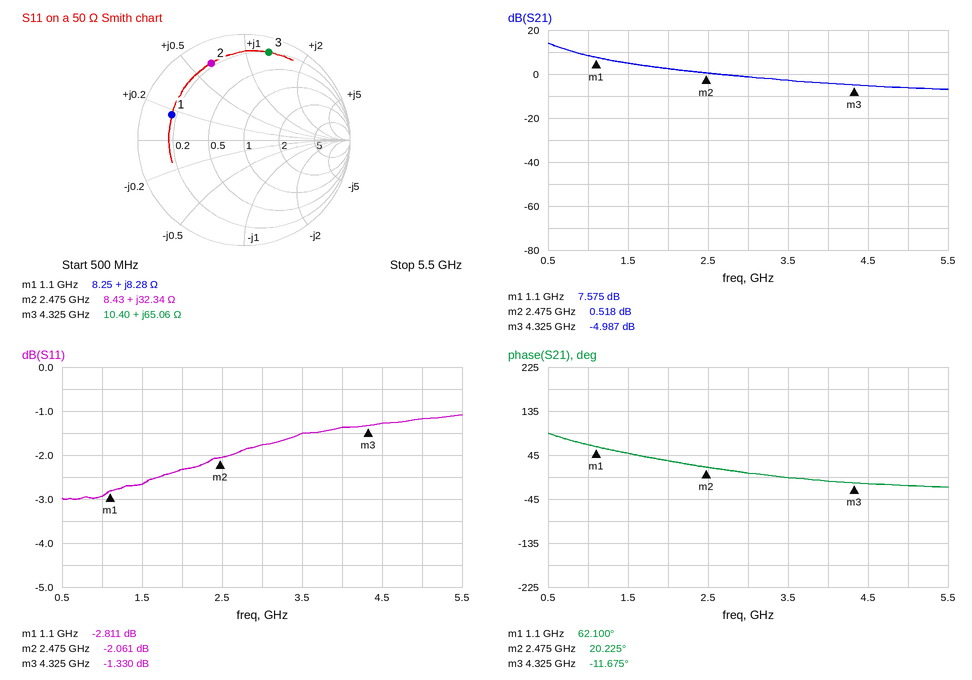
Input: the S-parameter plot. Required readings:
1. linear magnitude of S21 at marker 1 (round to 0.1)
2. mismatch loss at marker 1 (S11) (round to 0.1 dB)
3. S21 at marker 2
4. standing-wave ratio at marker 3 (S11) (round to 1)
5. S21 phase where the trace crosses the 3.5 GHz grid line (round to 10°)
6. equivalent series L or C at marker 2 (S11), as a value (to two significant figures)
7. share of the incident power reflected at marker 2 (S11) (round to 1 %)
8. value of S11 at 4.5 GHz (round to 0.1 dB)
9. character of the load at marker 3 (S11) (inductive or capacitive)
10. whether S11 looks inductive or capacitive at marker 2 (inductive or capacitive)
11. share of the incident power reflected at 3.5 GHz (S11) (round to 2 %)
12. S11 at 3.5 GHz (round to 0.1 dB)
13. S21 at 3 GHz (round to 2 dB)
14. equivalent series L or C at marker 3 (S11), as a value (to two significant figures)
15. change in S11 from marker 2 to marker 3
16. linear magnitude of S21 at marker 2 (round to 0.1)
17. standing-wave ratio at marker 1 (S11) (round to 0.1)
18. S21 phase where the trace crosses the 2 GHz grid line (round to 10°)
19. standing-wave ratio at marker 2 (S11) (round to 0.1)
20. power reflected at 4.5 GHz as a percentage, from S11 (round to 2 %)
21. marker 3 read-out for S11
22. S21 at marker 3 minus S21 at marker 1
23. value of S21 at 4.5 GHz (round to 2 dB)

2.4
3.2 dB
0.518 dB
13
0°
2.1 nH
62 %
-1.3 dB
inductive
inductive
70 %
-1.5 dB
-2 dB
2.4 nH
0.731 dB
1.1
6.2
30°
8.5
74 %
-1.330 dB
-12.562 dB
-6 dB
